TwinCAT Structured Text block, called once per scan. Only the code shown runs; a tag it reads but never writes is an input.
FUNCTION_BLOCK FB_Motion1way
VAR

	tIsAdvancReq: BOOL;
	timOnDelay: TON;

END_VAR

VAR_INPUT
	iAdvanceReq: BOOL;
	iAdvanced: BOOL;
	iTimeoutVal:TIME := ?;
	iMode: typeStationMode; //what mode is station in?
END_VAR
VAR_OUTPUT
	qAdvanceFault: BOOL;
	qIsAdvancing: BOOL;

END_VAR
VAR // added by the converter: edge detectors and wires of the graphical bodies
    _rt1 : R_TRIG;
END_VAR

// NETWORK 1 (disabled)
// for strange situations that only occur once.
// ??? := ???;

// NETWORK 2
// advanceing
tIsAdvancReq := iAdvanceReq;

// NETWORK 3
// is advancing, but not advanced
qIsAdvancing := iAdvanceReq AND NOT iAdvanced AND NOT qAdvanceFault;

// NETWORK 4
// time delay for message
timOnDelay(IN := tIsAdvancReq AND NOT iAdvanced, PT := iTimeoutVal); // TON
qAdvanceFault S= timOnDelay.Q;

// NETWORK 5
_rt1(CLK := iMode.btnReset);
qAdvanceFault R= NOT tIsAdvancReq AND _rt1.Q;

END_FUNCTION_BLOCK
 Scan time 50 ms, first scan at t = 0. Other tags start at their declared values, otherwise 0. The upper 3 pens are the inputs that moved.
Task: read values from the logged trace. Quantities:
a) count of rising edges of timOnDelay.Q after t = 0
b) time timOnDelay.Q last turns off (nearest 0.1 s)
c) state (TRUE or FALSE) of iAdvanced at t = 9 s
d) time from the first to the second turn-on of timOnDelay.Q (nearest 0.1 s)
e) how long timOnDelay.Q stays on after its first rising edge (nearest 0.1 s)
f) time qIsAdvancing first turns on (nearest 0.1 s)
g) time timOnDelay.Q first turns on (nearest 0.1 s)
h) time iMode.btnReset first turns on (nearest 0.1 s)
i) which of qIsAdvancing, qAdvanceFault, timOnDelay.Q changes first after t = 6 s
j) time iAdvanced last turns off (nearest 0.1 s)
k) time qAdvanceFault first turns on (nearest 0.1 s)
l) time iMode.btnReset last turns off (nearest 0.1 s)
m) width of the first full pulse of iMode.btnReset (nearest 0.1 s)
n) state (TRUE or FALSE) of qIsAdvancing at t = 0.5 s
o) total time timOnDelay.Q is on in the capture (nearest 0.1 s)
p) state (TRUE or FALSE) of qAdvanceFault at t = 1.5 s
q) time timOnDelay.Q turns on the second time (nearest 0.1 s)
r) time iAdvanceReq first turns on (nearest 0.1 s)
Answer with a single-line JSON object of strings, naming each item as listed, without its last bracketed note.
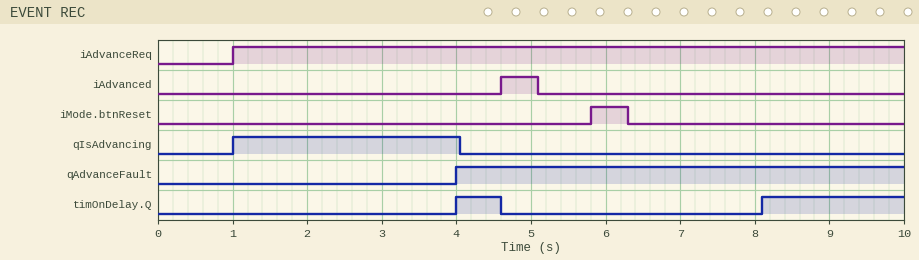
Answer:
{"count of rising edges of timOnDelay.Q after t = 0": "2", "time timOnDelay.Q last turns off": "4.6 s", "state (TRUE or FALSE) of iAdvanced at t = 9 s": "FALSE", "time from the first to the second turn-on of timOnDelay.Q": "4.1 s", "how long timOnDelay.Q stays on after its first rising edge": "0.6 s", "time qIsAdvancing first turns on": "1.0 s", "time timOnDelay.Q first turns on": "4.0 s", "time iMode.btnReset first turns on": "5.8 s", "which of qIsAdvancing, qAdvanceFault, timOnDelay.Q changes first after t = 6 s": "timOnDelay.Q", "time iAdvanced last turns off": "5.1 s", "time qAdvanceFault first turns on": "4.0 s", "time iMode.btnReset last turns off": "6.3 s", "width of the first full pulse of iMode.btnReset": "0.5 s", "state (TRUE or FALSE) of qIsAdvancing at t = 0.5 s": "FALSE", "total time timOnDelay.Q is on in the capture": "2.5 s", "state (TRUE or FALSE) of qAdvanceFault at t = 1.5 s": "FALSE", "time timOnDelay.Q turns on the second time": "8.1 s", "time iAdvanceReq first turns on": "1.0 s"}
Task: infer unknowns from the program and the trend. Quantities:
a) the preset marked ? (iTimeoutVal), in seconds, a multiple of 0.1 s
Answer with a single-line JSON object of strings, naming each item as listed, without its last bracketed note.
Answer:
{"the preset marked ? (iTimeoutVal), in seconds, a multiple of 0.1 s": "3.0 s"}
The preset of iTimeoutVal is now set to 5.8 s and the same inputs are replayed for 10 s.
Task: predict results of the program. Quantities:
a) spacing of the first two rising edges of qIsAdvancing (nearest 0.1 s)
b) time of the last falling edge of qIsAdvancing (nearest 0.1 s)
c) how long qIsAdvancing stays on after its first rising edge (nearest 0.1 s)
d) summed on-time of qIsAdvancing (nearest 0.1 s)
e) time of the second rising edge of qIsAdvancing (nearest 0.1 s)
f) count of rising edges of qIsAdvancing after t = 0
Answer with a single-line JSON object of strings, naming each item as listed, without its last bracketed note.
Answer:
{"spacing of the first two rising edges of qIsAdvancing": "4.1 s", "time of the last falling edge of qIsAdvancing": "4.6 s", "how long qIsAdvancing stays on after its first rising edge": "3.6 s", "summed on-time of qIsAdvancing": "8.5 s", "time of the second rising edge of qIsAdvancing": "5.1 s", "count of rising edges of qIsAdvancing after t = 0": "2"}
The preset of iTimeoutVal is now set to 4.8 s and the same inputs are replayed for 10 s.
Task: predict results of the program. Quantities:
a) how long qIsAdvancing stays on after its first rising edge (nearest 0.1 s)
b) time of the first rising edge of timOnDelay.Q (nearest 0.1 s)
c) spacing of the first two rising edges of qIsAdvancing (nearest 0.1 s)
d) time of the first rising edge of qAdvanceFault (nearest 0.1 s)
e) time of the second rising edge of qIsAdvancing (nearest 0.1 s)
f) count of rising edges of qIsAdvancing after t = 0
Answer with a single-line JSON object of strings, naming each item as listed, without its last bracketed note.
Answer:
{"how long qIsAdvancing stays on after its first rising edge": "3.6 s", "time of the first rising edge of timOnDelay.Q": "9.9 s", "spacing of the first two rising edges of qIsAdvancing": "4.1 s", "time of the first rising edge of qAdvanceFault": "9.9 s", "time of the second rising edge of qIsAdvancing": "5.1 s", "count of rising edges of qIsAdvancing after t = 0": "2"}
